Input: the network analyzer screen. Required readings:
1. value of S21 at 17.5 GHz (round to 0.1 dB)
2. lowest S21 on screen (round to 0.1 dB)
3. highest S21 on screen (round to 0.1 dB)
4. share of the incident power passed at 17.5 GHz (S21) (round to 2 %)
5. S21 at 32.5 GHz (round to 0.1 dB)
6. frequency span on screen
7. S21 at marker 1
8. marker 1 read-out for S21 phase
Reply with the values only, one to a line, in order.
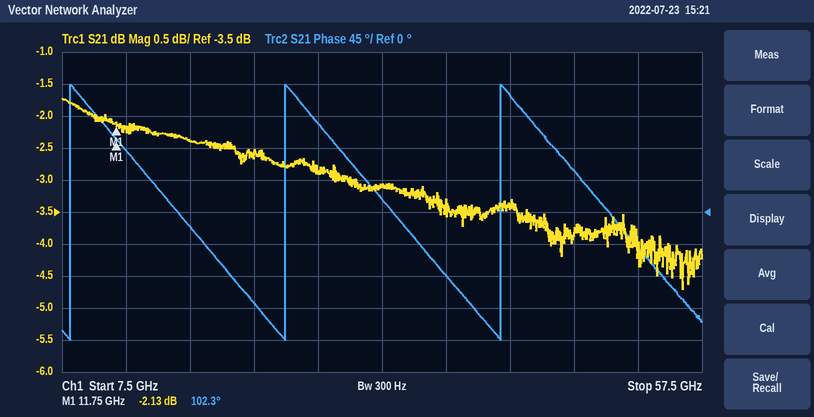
-2.4 dB
-4.7 dB
-1.7 dB
58 %
-3.1 dB
50 GHz
-2.13 dB
102.3°
